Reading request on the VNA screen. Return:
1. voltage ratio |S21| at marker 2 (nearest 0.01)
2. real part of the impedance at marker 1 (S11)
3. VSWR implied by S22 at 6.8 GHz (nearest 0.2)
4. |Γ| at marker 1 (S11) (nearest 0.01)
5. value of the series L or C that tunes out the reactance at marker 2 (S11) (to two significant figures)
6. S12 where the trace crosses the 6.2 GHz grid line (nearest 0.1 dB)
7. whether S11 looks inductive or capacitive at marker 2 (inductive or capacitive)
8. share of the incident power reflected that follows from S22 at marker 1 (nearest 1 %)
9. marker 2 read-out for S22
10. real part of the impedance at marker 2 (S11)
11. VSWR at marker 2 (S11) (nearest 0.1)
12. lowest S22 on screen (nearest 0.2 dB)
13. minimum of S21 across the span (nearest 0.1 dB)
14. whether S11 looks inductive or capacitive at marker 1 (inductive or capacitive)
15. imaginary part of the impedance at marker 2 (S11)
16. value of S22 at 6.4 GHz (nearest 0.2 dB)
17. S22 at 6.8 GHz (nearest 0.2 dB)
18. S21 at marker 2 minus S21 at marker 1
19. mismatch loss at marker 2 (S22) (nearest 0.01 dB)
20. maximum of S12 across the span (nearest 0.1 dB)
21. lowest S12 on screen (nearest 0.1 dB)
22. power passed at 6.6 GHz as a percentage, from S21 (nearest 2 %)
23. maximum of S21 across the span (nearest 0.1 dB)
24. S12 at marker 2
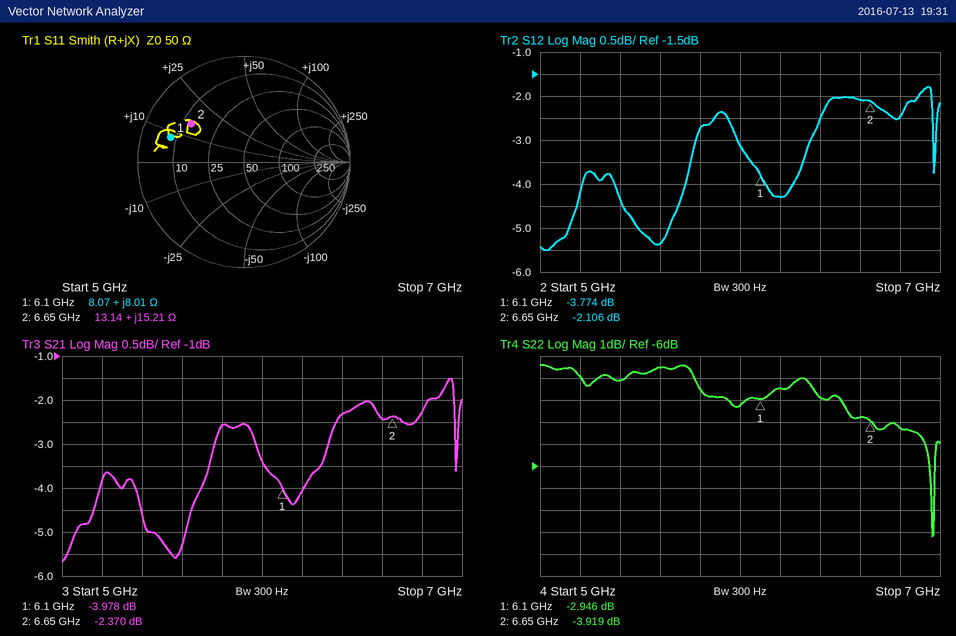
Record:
0.76
8.07 Ω
4.2
0.73
1.6 pF
-4.3 dB
inductive
51 %
-3.919 dB
13.14 Ω
4.2
-9.2 dB
-5.7 dB
inductive
+15.21 Ω
-2.8 dB
-4.2 dB
1.608 dB
2.26 dB
-1.8 dB
-5.5 dB
58 %
-1.5 dB
-2.106 dB
